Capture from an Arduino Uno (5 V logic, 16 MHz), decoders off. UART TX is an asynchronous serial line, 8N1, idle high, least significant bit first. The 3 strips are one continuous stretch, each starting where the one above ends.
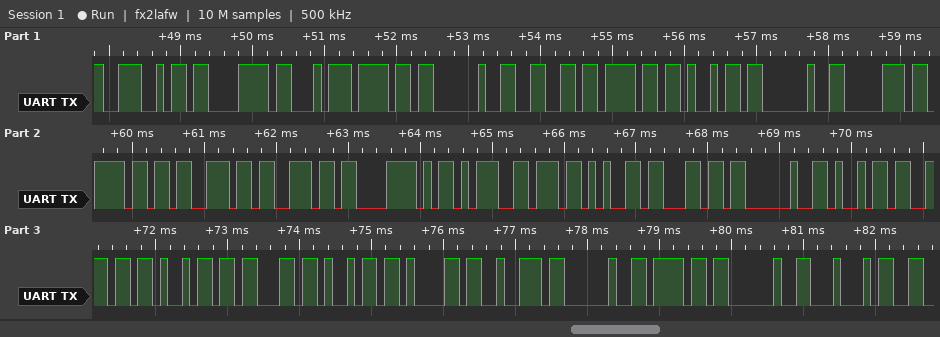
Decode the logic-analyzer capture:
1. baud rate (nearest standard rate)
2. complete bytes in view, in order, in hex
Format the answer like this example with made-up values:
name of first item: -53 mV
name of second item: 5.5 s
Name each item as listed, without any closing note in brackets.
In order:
baud rate: 9600 baud
complete bytes in view, in order, in hex: 4E C3 A3 6F 20 66 6F 69 20 70 6F 73 73 C3 AD 76 65 6C 20 69 6E 69 63 69 61 72 20 6F 20 44
